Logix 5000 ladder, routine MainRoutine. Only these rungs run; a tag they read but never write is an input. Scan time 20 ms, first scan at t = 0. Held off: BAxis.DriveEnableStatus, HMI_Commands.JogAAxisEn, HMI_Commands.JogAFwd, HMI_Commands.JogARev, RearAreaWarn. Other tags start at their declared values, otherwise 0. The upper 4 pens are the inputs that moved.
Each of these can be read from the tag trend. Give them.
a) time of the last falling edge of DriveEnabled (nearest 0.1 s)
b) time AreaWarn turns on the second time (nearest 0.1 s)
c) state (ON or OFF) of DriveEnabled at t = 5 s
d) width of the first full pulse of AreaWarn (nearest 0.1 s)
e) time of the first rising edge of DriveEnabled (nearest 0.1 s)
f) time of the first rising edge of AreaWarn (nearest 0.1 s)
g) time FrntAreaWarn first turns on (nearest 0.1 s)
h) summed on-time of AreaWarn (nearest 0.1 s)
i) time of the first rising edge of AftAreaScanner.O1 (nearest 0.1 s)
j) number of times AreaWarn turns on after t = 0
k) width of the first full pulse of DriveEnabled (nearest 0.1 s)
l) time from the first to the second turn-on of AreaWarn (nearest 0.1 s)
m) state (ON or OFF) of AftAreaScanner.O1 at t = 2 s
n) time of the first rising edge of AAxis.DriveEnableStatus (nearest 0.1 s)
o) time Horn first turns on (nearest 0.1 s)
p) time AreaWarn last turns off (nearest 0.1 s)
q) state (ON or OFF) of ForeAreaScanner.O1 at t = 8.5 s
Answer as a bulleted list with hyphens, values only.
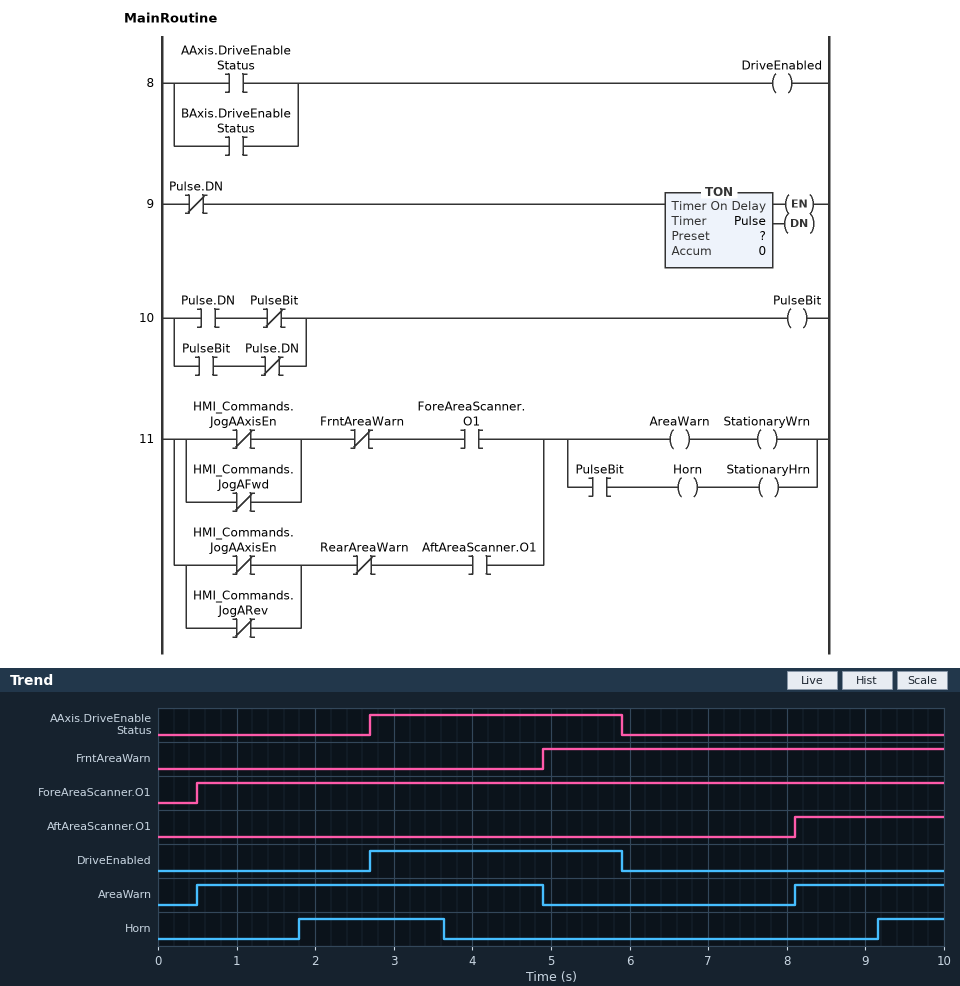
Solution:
- 5.9 s
- 8.1 s
- ON
- 4.4 s
- 2.7 s
- 0.5 s
- 4.9 s
- 6.3 s
- 8.1 s
- 2
- 3.2 s
- 7.6 s
- OFF
- 2.7 s
- 1.8 s
- 4.9 s
- ON
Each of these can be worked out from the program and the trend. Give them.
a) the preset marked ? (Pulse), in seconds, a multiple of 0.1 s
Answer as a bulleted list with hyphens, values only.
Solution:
- 1.8 s
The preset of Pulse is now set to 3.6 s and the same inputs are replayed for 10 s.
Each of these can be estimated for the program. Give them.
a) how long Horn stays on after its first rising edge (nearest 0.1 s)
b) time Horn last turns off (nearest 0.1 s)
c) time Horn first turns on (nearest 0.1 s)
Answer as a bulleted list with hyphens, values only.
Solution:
- 1.3 s
- 4.9 s
- 3.6 s
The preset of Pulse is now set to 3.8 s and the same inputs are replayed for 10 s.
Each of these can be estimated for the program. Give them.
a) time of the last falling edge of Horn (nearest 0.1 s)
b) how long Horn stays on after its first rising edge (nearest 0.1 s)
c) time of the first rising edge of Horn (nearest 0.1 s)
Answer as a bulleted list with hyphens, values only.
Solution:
- 4.9 s
- 1.1 s
- 3.8 s
